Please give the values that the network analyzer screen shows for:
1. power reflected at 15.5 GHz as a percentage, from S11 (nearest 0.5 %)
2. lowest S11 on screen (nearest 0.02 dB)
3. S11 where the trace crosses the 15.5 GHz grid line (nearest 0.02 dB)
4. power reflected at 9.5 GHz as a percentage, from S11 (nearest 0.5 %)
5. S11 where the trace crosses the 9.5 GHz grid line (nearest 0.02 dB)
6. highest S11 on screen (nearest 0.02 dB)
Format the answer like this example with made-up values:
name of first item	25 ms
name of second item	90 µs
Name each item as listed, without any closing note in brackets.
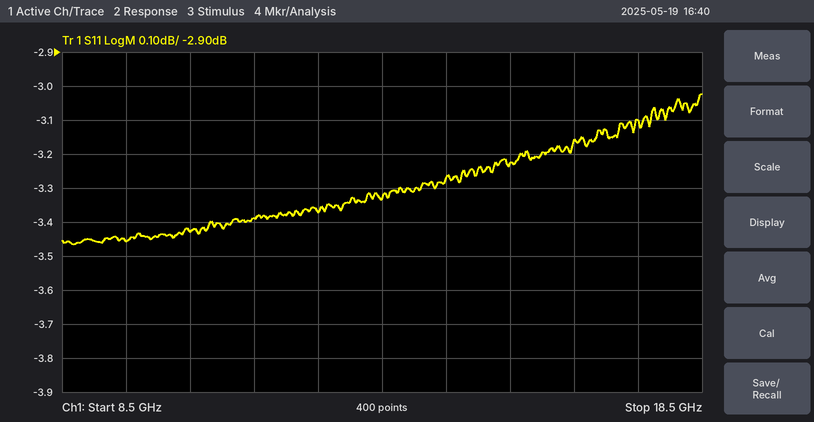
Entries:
power reflected at 15.5 GHz as a percentage, from S11	47.5 %
lowest S11 on screen	-3.46 dB
S11 where the trace crosses the 15.5 GHz grid line	-3.22 dB
power reflected at 9.5 GHz as a percentage, from S11	45.0 %
S11 where the trace crosses the 9.5 GHz grid line	-3.46 dB
highest S11 on screen	-3.02 dB
